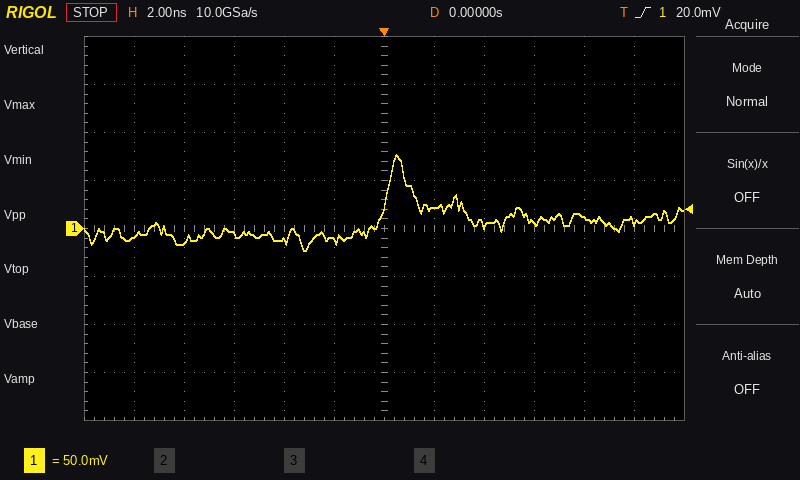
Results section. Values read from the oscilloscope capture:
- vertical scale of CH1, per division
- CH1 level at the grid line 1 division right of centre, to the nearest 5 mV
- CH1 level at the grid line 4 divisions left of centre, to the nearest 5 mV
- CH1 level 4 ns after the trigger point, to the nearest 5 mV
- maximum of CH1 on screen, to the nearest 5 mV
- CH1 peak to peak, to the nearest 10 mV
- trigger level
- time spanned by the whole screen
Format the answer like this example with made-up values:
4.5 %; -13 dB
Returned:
50 mV; 20 mV; -15 mV; 5 mV; 75 mV; 100 mV; 20.0 mV; 24 ns
